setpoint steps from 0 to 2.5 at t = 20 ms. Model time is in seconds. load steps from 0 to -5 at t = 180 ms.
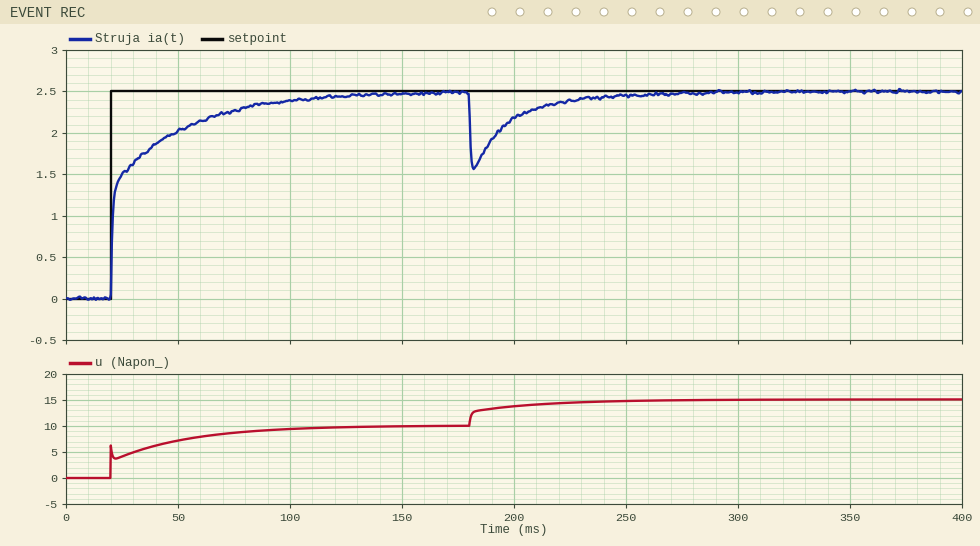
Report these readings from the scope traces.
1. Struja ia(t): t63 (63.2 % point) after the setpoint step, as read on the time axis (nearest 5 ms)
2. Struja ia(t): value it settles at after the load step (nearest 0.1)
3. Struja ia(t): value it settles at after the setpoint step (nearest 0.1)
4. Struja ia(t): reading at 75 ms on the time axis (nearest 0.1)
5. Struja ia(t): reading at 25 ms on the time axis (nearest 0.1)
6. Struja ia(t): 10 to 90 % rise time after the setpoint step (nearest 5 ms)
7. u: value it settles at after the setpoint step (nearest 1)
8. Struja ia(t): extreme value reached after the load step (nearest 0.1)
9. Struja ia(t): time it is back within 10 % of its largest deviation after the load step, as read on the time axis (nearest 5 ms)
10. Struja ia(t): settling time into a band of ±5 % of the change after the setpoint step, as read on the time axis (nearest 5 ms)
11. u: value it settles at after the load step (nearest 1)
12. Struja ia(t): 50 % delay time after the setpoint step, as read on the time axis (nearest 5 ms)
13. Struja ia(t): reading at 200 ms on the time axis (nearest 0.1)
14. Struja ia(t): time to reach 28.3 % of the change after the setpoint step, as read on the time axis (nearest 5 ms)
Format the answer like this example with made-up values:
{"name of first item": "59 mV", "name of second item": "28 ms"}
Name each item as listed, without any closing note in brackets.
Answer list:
{"Struja ia(t): t63 (63.2 % point) after the setpoint step, as read on the time axis": "30 ms", "Struja ia(t): value it settles at after the load step": "2.5", "Struja ia(t): value it settles at after the setpoint step": "2.5", "Struja ia(t): reading at 75 ms on the time axis": "2.3", "Struja ia(t): reading at 25 ms on the time axis": "1.5", "Struja ia(t): 10 to 90 % rise time after the setpoint step": "50 ms", "u: value it settles at after the setpoint step": "10", "Struja ia(t): extreme value reached after the load step": "1.6", "Struja ia(t): time it is back within 10 % of its largest deviation after the load step, as read on the time axis": "230 ms", "Struja ia(t): settling time into a band of ±5 % of the change after the setpoint step, as read on the time axis": "95 ms", "u: value it settles at after the load step": "15", "Struja ia(t): 50 % delay time after the setpoint step, as read on the time axis": "20 ms", "Struja ia(t): reading at 200 ms on the time axis": "2.2", "Struja ia(t): time to reach 28.3 % of the change after the setpoint step, as read on the time axis": "20 ms"}
